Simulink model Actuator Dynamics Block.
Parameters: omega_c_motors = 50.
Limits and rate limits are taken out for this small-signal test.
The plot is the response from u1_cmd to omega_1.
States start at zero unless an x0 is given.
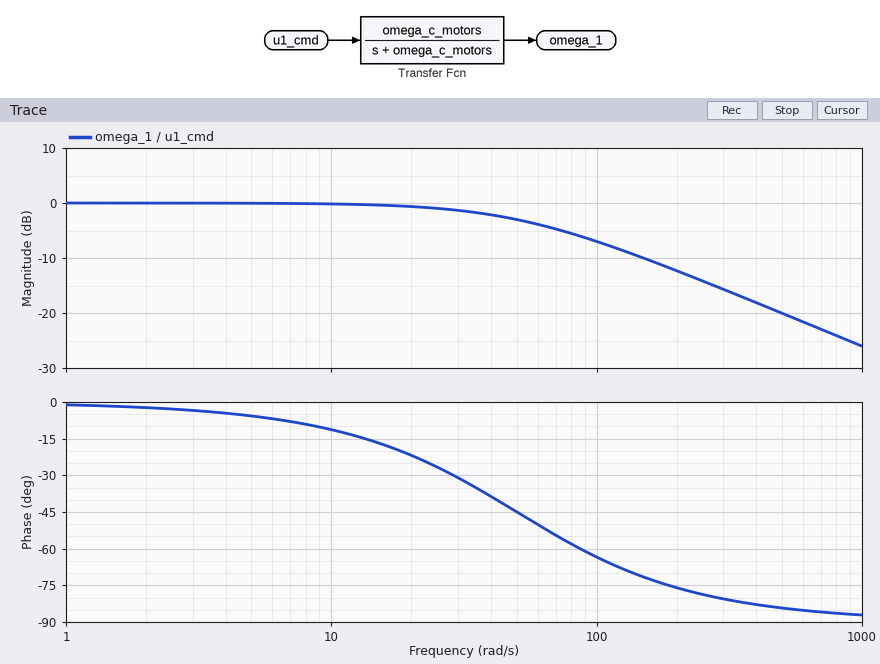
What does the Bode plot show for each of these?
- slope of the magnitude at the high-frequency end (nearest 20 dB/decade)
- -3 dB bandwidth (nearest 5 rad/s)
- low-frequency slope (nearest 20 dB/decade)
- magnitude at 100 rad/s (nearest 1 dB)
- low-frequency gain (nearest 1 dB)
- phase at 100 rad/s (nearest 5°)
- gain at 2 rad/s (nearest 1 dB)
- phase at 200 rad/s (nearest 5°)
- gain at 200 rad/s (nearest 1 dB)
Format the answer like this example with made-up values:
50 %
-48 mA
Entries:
-20 dB/decade
50 rad/s
0 dB/decade
-7 dB
0 dB
-65°
0 dB
-75°
-12 dB
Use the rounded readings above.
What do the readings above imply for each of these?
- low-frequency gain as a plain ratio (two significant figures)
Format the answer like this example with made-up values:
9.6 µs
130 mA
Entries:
1.0
